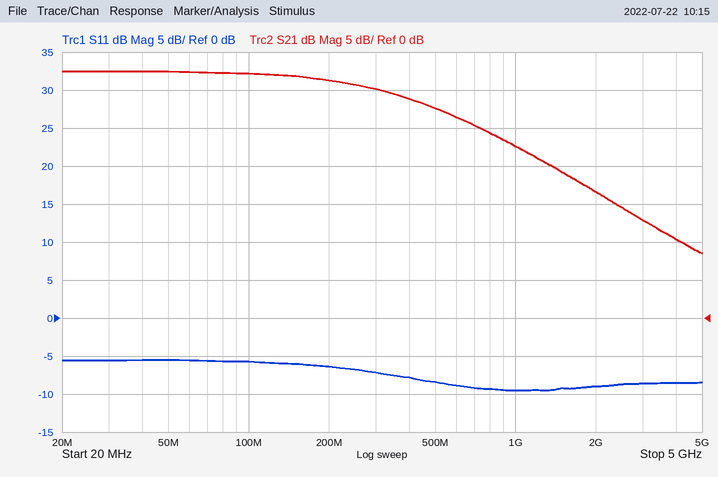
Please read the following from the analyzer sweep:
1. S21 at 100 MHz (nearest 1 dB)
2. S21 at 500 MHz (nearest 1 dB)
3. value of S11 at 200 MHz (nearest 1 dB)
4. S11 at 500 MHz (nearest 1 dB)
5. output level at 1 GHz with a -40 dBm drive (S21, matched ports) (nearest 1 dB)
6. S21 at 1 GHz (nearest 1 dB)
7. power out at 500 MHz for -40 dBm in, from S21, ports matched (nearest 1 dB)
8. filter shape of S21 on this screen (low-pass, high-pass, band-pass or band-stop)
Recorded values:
32 dB
28 dB
-6 dB
-8 dB
-17 dBm
23 dB
-12 dBm
low-pass
